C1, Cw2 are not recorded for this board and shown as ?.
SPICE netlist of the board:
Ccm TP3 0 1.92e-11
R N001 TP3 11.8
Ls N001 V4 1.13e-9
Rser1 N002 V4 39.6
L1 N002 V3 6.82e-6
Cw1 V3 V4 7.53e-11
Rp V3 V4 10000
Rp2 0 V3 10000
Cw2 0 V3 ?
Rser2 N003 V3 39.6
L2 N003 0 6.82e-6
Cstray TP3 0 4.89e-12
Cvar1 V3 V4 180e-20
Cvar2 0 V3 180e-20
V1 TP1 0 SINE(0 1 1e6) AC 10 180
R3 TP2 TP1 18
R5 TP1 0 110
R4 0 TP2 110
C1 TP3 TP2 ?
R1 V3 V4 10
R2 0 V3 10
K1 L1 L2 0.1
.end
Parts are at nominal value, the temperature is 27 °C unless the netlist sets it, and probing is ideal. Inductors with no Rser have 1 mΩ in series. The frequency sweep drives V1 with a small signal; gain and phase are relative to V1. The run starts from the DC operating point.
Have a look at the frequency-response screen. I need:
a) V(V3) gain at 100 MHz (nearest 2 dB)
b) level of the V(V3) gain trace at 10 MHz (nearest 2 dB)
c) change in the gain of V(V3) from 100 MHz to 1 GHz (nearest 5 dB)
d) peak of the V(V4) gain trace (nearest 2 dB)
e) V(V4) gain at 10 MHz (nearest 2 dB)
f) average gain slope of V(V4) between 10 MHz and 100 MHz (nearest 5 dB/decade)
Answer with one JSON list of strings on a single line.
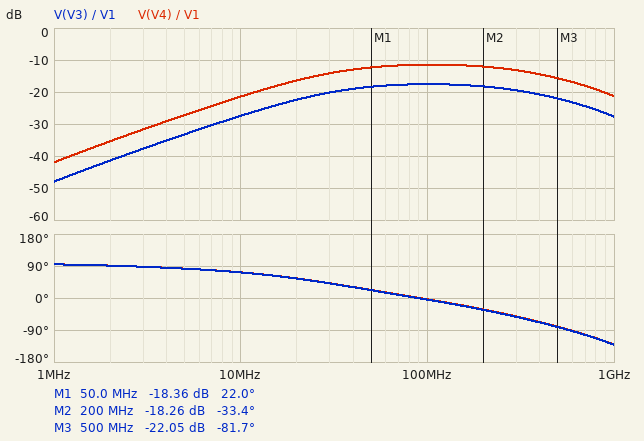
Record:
["-18 dB", "-28 dB", "-10 dB", "-12 dB", "-22 dB", "10 dB/decade"]
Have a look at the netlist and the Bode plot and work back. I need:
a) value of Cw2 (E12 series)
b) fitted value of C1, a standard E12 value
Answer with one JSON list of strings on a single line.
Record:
["82 pF", "82 pF"]
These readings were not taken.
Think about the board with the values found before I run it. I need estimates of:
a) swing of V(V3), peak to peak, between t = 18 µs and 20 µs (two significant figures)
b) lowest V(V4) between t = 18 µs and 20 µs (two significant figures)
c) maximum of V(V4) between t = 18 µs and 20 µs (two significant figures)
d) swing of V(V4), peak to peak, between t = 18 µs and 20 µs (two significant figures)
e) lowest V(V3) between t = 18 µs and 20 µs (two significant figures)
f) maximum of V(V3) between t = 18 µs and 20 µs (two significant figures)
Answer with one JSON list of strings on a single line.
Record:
["8.0 mV", "-8.0 mV", "8.0 mV", "16 mV", "-4.0 mV", "4.0 mV"]
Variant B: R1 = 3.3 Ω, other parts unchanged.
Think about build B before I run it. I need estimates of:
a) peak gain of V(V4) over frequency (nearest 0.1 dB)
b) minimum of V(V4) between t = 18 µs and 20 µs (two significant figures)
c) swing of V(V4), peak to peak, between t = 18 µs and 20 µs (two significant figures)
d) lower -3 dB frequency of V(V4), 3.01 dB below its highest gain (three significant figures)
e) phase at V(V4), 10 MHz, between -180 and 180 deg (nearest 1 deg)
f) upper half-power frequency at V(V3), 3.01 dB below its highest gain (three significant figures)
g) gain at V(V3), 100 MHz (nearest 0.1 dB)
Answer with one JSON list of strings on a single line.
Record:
["-13.6 dB", "-5.4 mV", "11 mV", "32.3 MHz", "75 deg", "330 MHz", "-16.3 dB"]
